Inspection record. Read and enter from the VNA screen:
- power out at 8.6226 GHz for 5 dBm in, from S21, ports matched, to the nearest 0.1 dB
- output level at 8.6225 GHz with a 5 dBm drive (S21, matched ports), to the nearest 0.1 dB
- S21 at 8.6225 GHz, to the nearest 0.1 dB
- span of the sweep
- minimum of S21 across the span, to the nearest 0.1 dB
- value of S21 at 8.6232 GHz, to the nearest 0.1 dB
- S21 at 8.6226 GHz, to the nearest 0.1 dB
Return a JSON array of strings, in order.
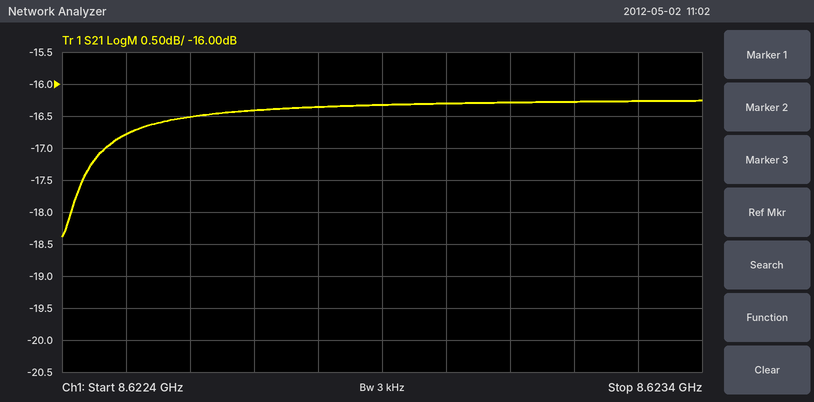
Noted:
["-11.5 dBm", "-11.8 dBm", "-16.8 dB", "1 MHz", "-18.4 dB", "-16.3 dB", "-16.5 dB"]
